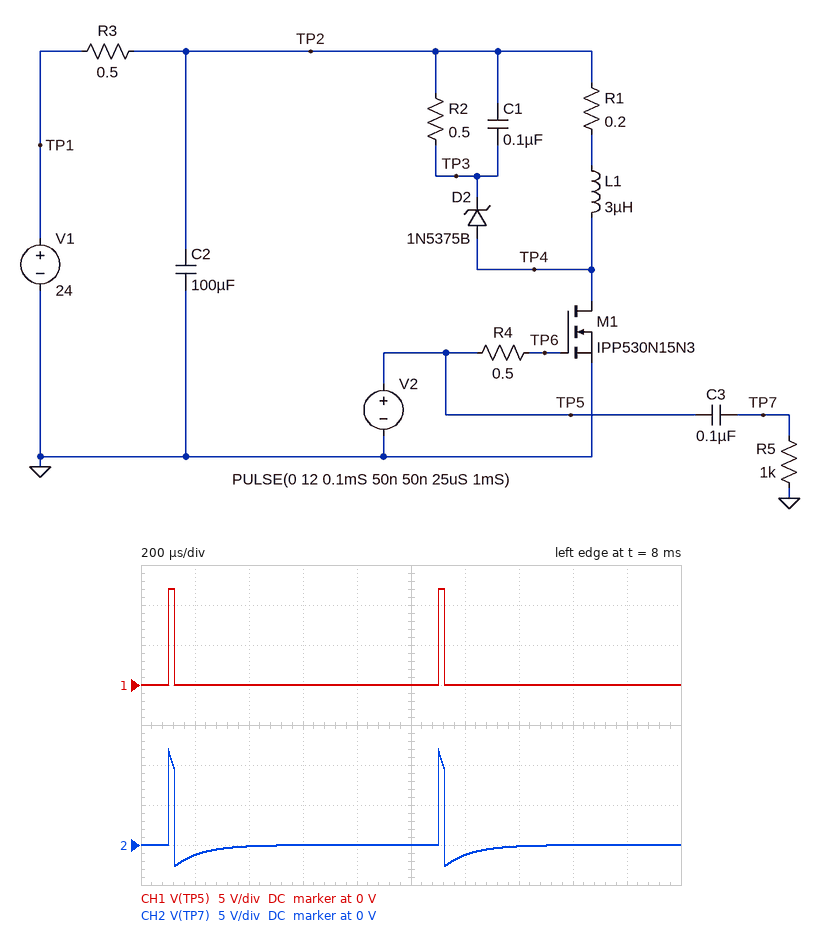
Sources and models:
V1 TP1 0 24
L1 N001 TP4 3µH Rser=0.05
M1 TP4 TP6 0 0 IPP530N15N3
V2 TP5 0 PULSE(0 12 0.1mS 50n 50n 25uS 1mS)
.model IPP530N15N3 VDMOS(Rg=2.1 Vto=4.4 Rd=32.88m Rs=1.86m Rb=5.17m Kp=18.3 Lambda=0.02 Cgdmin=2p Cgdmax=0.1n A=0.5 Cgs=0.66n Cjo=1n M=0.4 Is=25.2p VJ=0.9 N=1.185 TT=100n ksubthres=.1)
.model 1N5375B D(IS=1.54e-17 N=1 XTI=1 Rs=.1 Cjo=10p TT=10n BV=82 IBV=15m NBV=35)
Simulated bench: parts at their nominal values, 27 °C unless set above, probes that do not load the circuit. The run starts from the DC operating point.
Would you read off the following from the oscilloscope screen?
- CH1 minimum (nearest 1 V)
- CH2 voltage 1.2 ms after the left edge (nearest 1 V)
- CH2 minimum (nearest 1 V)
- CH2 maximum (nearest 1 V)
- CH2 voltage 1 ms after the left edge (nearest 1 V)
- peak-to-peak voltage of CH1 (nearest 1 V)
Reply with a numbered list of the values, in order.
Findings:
1. 0 V
2. -1 V
3. -3 V
4. 12 V
5. 0 V
6. 12 V
